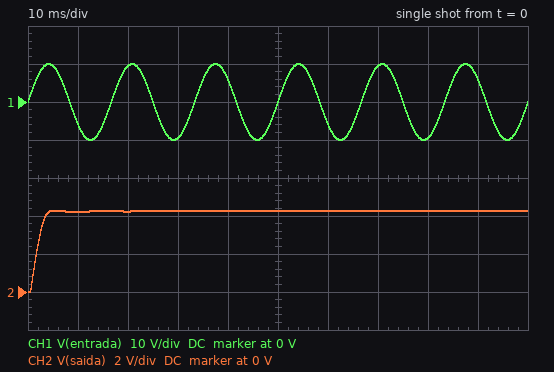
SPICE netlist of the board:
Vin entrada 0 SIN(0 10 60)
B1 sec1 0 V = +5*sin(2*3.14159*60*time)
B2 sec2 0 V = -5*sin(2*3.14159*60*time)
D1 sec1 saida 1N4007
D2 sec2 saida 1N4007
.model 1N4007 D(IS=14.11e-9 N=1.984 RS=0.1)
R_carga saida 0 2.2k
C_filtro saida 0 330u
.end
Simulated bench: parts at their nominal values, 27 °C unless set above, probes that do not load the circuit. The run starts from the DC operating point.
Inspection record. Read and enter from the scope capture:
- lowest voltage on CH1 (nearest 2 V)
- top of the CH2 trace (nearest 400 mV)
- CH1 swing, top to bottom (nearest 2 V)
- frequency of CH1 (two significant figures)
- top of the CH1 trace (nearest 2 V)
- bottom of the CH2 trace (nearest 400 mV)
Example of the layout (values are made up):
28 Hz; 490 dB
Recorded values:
-10 V; 4.4 V; 20 V; 60 Hz; 10 V; 0 V
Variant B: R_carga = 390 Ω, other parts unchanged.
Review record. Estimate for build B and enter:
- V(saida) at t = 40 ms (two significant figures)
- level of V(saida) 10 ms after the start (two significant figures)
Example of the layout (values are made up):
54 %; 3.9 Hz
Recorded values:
4.2 V; 4.1 V
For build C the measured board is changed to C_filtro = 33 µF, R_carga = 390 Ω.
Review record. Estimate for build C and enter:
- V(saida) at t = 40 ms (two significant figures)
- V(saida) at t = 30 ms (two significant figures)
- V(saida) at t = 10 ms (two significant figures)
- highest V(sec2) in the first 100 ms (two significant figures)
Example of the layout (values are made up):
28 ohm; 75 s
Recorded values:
3.7 V; 4.2 V; 2.8 V; 5.0 V
